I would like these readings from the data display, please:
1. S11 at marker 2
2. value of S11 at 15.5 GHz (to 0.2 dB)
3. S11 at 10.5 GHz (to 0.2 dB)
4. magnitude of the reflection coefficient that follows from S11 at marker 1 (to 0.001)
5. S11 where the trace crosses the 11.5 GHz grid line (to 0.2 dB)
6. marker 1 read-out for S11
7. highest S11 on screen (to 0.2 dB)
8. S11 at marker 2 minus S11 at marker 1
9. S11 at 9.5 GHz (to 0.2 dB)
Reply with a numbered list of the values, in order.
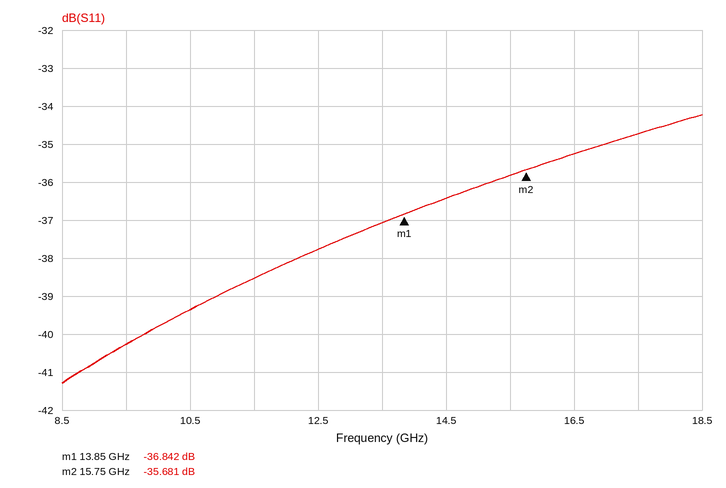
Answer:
1. -35.681 dB
2. -35.8 dB
3. -39.4 dB
4. 0.014
5. -38.6 dB
6. -36.842 dB
7. -34.2 dB
8. 1.161 dB
9. -40.2 dB
